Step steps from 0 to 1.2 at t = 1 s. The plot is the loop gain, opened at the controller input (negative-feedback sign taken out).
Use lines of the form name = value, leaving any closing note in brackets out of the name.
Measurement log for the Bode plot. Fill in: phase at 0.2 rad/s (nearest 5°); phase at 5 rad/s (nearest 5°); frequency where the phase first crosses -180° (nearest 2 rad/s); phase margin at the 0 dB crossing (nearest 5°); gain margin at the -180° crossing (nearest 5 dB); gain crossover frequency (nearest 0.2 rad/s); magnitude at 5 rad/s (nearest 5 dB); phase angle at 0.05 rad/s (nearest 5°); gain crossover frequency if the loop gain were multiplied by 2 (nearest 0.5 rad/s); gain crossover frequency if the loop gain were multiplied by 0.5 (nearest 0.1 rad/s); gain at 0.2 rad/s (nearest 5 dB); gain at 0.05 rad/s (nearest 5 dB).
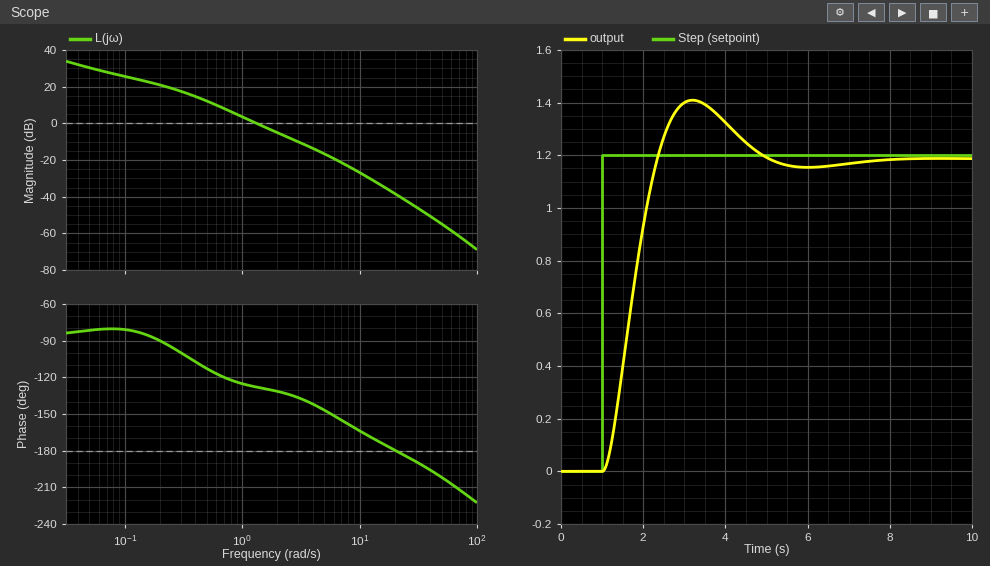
phase at 0.2 rad/s = -90°
phase at 5 rad/s = -145°
frequency where the phase first crosses -180° = 20 rad/s
phase margin at the 0 dB crossing = 50°
gain margin at the -180° crossing = 40 dB
gain crossover frequency = 1.4 rad/s
magnitude at 5 rad/s = -15 dB
phase angle at 0.05 rad/s = -80°
gain crossover frequency if the loop gain were multiplied by 2 = 2.0 rad/s
gain crossover frequency if the loop gain were multiplied by 0.5 = 0.8 rad/s
gain at 0.2 rad/s = 20 dB
gain at 0.05 rad/s = 30 dB
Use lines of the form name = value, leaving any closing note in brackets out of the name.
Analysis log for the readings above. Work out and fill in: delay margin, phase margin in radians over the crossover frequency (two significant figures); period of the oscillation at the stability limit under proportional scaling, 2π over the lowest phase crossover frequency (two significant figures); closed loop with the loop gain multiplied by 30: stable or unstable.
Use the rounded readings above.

delay margin, phase margin in radians over the crossover frequency = 0.62 s
period of the oscillation at the stability limit under proportional scaling, 2π over the lowest phase crossover frequency = 0.31 s
closed loop with the loop gain multiplied by 30: stable or unstable = stable
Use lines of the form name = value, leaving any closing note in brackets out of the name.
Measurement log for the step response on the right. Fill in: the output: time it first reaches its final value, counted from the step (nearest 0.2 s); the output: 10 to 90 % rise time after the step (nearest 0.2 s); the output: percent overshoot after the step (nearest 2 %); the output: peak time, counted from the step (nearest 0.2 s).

the output: time it first reaches its final value, counted from the step = 1.4 s
the output: 10 to 90 % rise time after the step = 1.0 s
the output: percent overshoot after the step = 18 %
the output: peak time, counted from the step = 2.2 s
